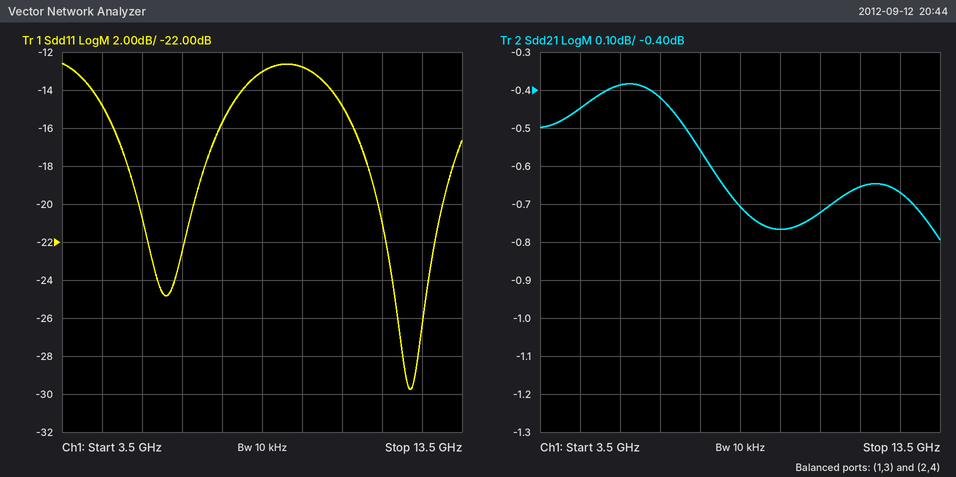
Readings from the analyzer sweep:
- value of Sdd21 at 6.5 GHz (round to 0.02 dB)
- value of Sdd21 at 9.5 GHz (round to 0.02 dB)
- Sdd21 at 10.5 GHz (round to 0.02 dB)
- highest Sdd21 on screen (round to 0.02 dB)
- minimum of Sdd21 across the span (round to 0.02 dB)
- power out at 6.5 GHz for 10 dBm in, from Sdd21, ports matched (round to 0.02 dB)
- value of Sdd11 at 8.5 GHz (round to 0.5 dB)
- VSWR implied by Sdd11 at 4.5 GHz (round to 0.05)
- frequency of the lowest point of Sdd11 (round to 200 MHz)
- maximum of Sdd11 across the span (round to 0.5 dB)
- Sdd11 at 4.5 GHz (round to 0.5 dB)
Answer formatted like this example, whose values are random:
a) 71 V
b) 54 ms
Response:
a) -0.42 dB
b) -0.76 dB
c) -0.72 dB
d) -0.38 dB
e) -0.80 dB
f) 9.58 dBm
g) -13.0 dB
h) 1.45
i) 12.2 GHz
j) -12.5 dB
k) -15.0 dB
